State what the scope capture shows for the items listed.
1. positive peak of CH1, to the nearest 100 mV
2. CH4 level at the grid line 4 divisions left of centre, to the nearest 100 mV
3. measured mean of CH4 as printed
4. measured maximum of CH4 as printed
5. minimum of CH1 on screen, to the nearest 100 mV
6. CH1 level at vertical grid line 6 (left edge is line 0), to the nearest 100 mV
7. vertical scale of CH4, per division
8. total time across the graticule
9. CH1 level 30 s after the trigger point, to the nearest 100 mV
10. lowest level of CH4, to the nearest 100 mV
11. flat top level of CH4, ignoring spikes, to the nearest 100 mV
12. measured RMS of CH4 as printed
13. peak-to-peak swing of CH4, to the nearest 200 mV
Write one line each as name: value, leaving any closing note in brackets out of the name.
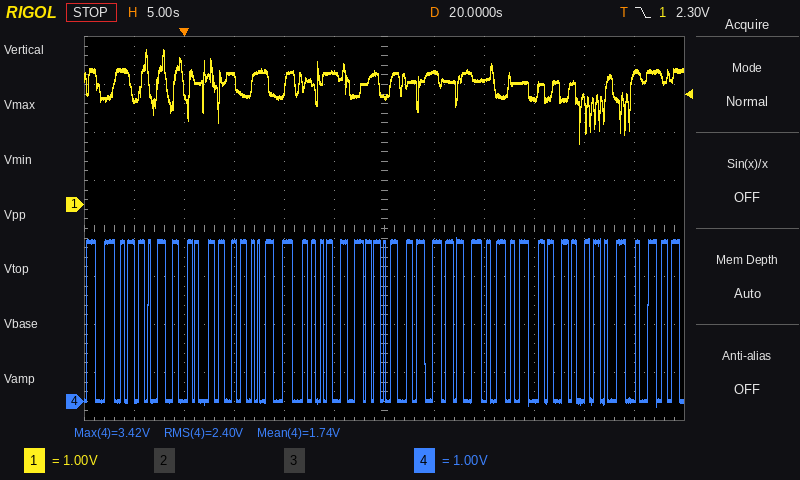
positive peak of CH1, to the nearest 100 mV: 3.2 V
CH4 level at the grid line 4 divisions left of centre, to the nearest 100 mV: 0.0 V
measured mean of CH4 as printed: 1.74 V
measured maximum of CH4 as printed: 3.42 V
minimum of CH1 on screen, to the nearest 100 mV: 1.3 V
CH1 level at vertical grid line 6 (left edge is line 0), to the nearest 100 mV: 2.2 V
vertical scale of CH4, per division: 1 V
total time across the graticule: 60 s
CH1 level 30 s after the trigger point, to the nearest 100 mV: 2.6 V
lowest level of CH4, to the nearest 100 mV: -100 mV
flat top level of CH4, ignoring spikes, to the nearest 100 mV: 3.3 V
measured RMS of CH4 as printed: 2.40 V
peak-to-peak swing of CH4, to the nearest 200 mV: 3.6 V
